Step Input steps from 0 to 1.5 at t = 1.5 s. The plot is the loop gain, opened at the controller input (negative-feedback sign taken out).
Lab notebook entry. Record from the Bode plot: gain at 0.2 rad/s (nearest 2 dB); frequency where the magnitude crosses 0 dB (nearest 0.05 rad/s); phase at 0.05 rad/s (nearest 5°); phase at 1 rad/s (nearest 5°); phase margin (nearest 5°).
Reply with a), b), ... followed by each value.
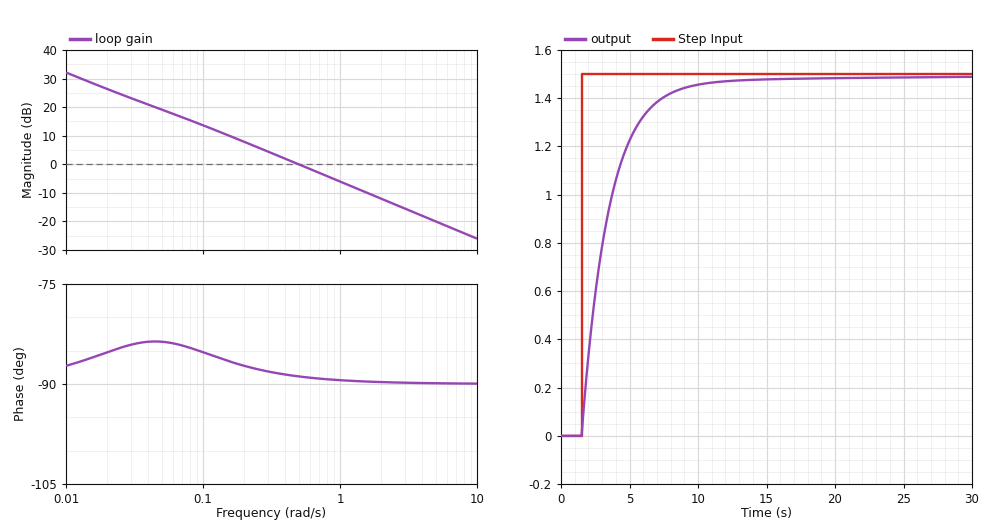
a) 8 dB
b) 0.50 rad/s
c) -85°
d) -90°
e) 90°
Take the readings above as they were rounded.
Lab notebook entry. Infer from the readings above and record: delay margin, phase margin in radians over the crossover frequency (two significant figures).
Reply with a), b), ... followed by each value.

a) 3.1 s
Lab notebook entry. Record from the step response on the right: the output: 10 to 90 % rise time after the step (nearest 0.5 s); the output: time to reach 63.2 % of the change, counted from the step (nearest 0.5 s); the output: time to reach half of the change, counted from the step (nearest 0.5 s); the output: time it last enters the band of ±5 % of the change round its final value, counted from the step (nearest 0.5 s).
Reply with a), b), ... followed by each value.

a) 4.5 s
b) 2.0 s
c) 1.5 s
d) 6.5 s
